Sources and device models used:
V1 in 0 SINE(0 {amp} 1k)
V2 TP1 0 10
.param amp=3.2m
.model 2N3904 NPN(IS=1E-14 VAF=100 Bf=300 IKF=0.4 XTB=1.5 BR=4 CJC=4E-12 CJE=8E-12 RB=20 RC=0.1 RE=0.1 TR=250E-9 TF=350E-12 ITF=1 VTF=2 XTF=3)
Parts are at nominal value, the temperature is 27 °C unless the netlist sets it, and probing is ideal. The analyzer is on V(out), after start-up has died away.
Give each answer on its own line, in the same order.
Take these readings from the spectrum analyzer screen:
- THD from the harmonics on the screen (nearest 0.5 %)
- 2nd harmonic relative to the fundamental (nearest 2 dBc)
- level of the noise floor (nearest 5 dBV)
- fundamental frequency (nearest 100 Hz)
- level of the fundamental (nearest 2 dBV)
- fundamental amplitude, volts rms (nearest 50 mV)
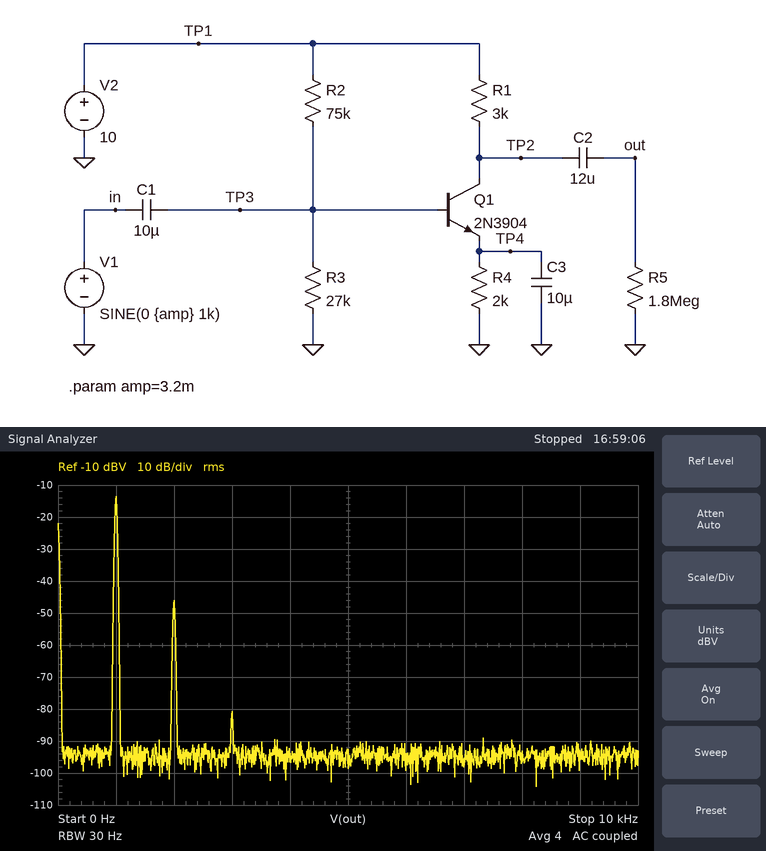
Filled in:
2.5 %
-32 dBc
-95 dBV
1.0 kHz
-14 dBV
200 mV
